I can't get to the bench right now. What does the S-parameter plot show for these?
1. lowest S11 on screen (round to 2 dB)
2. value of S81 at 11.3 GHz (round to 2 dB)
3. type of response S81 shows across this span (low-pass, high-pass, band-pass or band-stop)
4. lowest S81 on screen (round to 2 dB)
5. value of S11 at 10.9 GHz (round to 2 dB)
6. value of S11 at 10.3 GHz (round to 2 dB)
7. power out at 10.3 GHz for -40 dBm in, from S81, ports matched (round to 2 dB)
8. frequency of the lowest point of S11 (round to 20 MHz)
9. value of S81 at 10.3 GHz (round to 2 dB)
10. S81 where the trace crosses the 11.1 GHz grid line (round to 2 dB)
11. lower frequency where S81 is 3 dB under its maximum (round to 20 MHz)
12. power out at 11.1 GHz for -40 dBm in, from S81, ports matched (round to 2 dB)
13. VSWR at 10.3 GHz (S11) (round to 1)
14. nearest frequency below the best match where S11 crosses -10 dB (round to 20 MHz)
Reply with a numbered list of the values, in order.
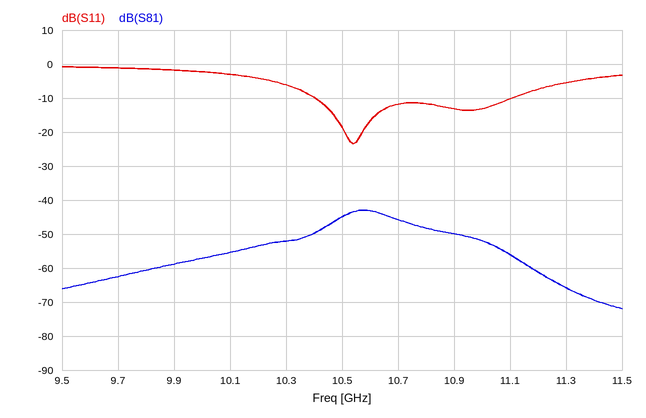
1. -24 dB
2. -66 dB
3. band-pass
4. -72 dB
5. -14 dB
6. -6 dB
7. -92 dBm
8. 10.54 GHz
9. -52 dB
10. -56 dB
11. 10.48 GHz
12. -96 dBm
13. 3
14. 10.40 GHz
